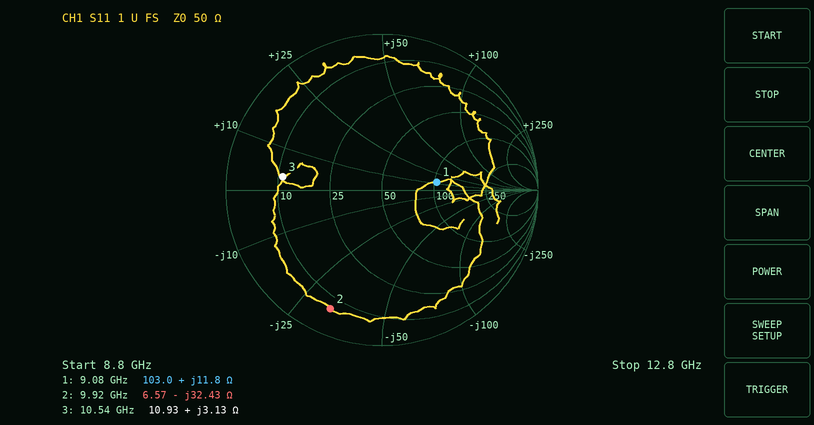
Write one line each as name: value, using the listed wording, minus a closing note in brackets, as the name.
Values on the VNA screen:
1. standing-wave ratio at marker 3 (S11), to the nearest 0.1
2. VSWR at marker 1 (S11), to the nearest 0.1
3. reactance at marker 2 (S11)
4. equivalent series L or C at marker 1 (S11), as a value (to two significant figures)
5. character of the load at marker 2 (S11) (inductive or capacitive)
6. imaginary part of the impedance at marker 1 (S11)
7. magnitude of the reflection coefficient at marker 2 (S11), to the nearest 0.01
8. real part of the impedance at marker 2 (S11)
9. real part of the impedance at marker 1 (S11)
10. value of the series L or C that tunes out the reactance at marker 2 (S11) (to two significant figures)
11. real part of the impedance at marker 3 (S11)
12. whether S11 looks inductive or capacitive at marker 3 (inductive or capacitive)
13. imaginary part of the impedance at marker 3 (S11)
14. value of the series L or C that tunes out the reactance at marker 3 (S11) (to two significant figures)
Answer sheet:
standing-wave ratio at marker 3 (S11), to the nearest 0.1: 4.6
VSWR at marker 1 (S11), to the nearest 0.1: 2.1
reactance at marker 2: -32.43 Ω
equivalent series L or C at marker 1 (S11), as a value: 210 pH
character of the load at marker 2 (S11): capacitive
imaginary part of the impedance at marker 1: +11.8 Ω
magnitude of the reflection coefficient at marker 2 (S11), to the nearest 0.01: 0.83
real part of the impedance at marker 2: 6.57 Ω
real part of the impedance at marker 1: 103.0 Ω
value of the series L or C that tunes out the reactance at marker 2 (S11): 520 pH
real part of the impedance at marker 3: 10.93 Ω
whether S11 looks inductive or capacitive at marker 3: inductive
imaginary part of the impedance at marker 3: +3.13 Ω
value of the series L or C that tunes out the reactance at marker 3 (S11): 4.8 pF
